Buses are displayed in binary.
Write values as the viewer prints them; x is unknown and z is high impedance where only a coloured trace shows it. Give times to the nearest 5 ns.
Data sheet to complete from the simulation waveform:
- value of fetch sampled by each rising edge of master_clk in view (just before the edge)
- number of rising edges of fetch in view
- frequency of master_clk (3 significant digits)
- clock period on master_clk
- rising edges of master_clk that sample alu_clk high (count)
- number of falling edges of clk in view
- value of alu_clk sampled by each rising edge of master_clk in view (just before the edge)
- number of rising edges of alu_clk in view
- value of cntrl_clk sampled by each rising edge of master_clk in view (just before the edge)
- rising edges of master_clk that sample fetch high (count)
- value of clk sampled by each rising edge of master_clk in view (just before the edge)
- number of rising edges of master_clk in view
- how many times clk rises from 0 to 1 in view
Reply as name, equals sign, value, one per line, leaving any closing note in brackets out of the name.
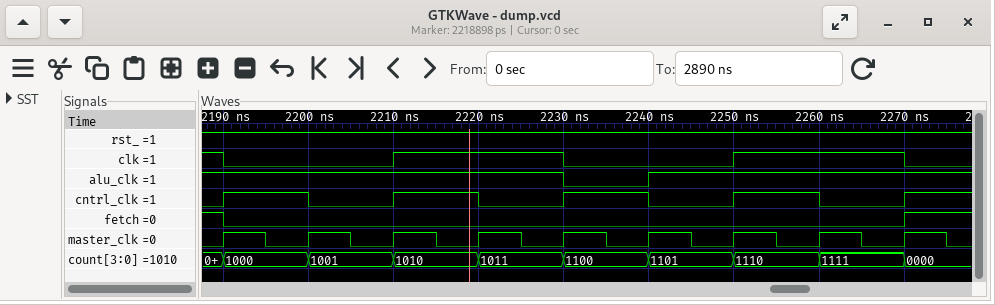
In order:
value of fetch sampled by each rising edge of master_clk in view = 1 0 0 0 0 0 0 0 0
number of rising edges of fetch in view = 1
frequency of master_clk = 100 MHz
clock period on master_clk = 10 ns
rising edges of master_clk that sample alu_clk high = 8
number of falling edges of clk in view = 3
value of alu_clk sampled by each rising edge of master_clk in view = 1 1 1 1 1 0 1 1 1
number of rising edges of alu_clk in view = 1
value of cntrl_clk sampled by each rising edge of master_clk in view = 0 1 0 1 0 1 0 1 0
rising edges of master_clk that sample fetch high = 1
value of clk sampled by each rising edge of master_clk in view = 1 0 0 1 1 0 0 1 1
number of rising edges of master_clk in view = 9
how many times clk rises from 0 to 1 in view = 2
